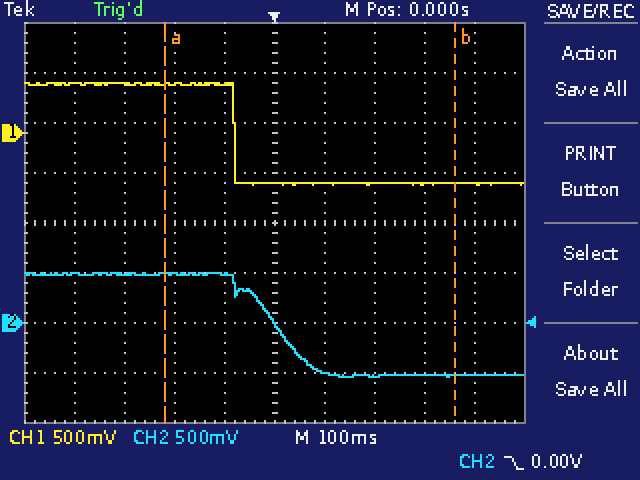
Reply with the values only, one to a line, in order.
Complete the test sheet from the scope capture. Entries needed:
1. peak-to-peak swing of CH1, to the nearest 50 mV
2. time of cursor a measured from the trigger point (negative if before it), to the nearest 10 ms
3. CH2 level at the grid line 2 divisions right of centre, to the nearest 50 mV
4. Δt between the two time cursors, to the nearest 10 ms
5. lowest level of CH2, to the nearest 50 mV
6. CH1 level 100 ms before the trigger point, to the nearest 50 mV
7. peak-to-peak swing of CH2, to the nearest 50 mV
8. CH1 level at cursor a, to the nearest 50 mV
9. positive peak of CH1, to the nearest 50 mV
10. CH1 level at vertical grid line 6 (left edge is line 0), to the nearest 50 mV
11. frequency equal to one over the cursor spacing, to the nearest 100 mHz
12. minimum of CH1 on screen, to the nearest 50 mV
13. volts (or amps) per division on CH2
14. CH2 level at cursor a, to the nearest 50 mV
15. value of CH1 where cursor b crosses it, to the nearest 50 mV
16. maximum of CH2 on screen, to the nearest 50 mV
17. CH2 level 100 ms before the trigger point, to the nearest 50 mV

1.00 V
-220 ms
-550 mV
580 ms
-550 mV
500 mV
1.05 V
500 mV
500 mV
-500 mV
1.7 Hz
-500 mV
500 mV
500 mV
-500 mV
500 mV
500 mV
